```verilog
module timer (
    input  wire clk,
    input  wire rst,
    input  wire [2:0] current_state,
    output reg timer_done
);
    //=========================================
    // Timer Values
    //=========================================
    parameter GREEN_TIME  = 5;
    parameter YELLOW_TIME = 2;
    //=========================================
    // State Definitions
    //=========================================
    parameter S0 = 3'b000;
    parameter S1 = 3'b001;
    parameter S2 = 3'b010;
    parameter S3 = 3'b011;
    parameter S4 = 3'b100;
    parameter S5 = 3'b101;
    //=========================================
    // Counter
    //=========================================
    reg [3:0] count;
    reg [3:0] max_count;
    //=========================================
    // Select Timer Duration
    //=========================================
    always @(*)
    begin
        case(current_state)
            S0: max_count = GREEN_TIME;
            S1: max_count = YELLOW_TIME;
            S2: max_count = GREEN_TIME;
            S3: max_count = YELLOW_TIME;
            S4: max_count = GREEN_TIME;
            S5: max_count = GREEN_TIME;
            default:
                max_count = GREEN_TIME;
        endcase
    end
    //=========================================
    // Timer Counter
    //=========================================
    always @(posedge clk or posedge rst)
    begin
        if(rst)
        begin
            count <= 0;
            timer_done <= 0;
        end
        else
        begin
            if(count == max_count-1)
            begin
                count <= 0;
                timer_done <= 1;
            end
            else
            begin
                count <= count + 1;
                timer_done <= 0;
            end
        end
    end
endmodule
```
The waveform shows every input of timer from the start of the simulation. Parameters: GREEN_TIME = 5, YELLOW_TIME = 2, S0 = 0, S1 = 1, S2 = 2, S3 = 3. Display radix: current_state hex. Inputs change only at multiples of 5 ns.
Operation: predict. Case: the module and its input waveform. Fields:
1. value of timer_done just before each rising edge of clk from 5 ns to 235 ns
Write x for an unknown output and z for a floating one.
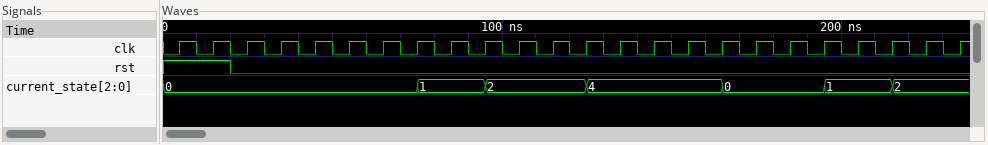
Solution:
0 0 0 0 0 0 0 1 0 1 0 0 0 0 1 0 0 0 0 1 0 1 0 0
